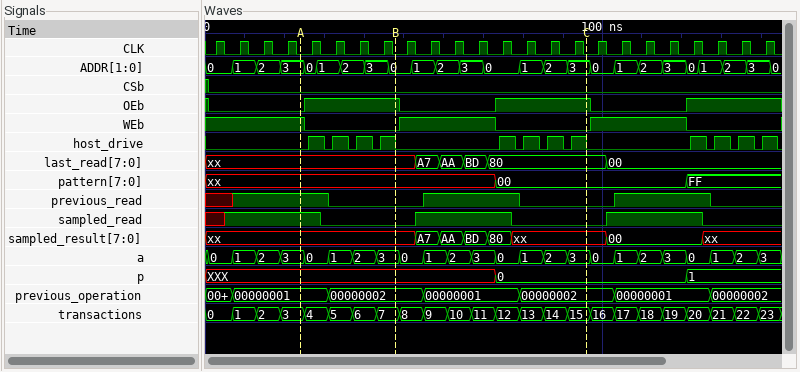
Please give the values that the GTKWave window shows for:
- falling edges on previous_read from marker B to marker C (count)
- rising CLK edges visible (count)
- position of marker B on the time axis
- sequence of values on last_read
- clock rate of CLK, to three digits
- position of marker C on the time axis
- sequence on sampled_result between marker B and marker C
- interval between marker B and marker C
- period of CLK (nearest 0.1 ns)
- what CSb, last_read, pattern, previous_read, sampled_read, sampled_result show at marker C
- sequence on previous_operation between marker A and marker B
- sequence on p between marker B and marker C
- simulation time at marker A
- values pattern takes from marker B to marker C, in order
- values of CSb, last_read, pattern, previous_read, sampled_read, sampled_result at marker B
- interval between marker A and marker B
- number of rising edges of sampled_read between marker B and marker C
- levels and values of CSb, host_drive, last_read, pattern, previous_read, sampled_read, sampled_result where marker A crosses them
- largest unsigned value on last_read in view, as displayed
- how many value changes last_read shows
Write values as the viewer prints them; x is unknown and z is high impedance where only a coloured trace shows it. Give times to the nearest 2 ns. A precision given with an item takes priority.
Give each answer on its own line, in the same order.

1
24
48 ns
xx, A7, AA, BD, 80, 00
167 MHz
96 ns
xx, A7, AA, BD, 80, xx
48 ns
6 ns
CSb=0, last_read=80, pattern=00, previous_read=0, sampled_read=0, sampled_result=xx
00000001, 00000002
XXX, 0
24 ns
xx, 00
CSb=0, last_read=xx, pattern=xx, previous_read=0, sampled_read=0, sampled_result=xx
24 ns
1
CSb=0, host_drive=0, last_read=xx, pattern=xx, previous_read=1, sampled_read=1, sampled_result=xx
BD
5
